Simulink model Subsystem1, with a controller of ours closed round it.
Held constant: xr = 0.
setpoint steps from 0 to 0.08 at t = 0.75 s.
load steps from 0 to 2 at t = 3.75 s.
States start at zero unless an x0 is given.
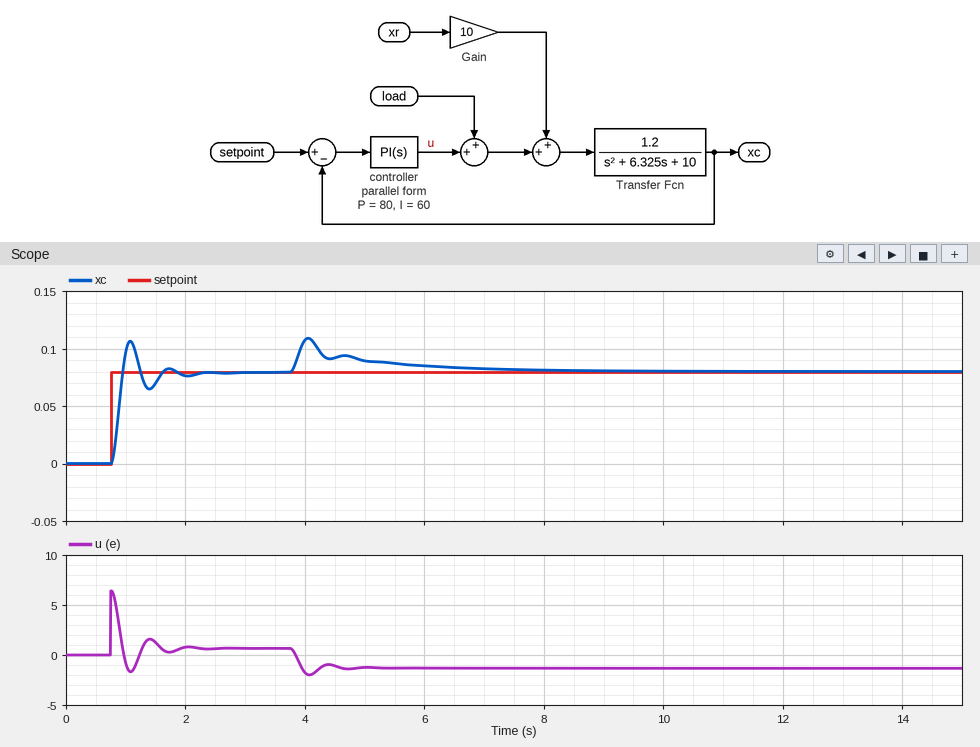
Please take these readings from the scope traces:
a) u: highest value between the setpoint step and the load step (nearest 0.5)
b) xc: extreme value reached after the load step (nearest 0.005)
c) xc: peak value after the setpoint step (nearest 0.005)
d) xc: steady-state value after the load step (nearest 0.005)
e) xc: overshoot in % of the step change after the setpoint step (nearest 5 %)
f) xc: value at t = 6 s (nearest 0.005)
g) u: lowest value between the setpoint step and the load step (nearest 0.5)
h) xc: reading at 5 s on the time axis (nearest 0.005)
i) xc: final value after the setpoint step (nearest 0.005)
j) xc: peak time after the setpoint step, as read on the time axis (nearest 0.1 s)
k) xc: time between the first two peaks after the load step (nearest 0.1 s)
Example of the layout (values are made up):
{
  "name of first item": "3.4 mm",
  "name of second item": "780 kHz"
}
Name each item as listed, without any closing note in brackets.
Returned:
{
  "u: highest value between the setpoint step and the load step": "6.5",
  "xc: extreme value reached after the load step": "0.110",
  "xc: peak value after the setpoint step": "0.105",
  "xc: steady-state value after the load step": "0.080",
  "xc: overshoot in % of the step change after the setpoint step": "35 %",
  "xc: value at t = 6 s": "0.085",
  "u: lowest value between the setpoint step and the load step": "-1.5",
  "xc: reading at 5 s on the time axis": "0.090",
  "xc: final value after the setpoint step": "0.080",
  "xc: peak time after the setpoint step, as read on the time axis": "1.1 s",
  "xc: time between the first two peaks after the load step": "0.6 s"
}
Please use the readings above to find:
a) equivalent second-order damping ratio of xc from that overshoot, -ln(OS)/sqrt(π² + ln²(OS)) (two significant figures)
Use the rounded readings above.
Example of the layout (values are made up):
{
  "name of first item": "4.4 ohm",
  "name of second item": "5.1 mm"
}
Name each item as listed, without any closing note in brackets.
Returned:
{
  "equivalent second-order damping ratio of xc from that overshoot, -ln(OS)/sqrt(π² + ln²(OS))": "0.32"
}
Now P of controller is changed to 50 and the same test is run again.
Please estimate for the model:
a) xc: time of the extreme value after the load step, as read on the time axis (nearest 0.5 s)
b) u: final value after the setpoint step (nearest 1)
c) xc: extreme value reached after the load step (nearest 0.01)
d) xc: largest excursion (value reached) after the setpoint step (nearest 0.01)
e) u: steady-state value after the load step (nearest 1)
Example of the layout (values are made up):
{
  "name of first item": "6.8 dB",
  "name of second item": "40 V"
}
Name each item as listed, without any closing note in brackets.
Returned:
{
  "xc: time of the extreme value after the load step, as read on the time axis": "4.0 s",
  "u: final value after the setpoint step": "1",
  "xc: extreme value reached after the load step": "0.12",
  "xc: largest excursion (value reached) after the setpoint step": "0.10",
  "u: steady-state value after the load step": "-1"
}
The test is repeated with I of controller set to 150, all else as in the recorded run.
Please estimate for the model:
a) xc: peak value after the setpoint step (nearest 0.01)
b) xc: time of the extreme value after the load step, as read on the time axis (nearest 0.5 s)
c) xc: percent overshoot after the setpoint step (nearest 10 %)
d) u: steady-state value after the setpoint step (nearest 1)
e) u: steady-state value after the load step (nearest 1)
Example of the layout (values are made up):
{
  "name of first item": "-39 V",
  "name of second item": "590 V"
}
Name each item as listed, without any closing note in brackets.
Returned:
{
  "xc: peak value after the setpoint step": "0.12",
  "xc: time of the extreme value after the load step, as read on the time axis": "4.0 s",
  "xc: percent overshoot after the setpoint step": "50 %",
  "u: steady-state value after the setpoint step": "1",
  "u: steady-state value after the load step": "-1"
}
